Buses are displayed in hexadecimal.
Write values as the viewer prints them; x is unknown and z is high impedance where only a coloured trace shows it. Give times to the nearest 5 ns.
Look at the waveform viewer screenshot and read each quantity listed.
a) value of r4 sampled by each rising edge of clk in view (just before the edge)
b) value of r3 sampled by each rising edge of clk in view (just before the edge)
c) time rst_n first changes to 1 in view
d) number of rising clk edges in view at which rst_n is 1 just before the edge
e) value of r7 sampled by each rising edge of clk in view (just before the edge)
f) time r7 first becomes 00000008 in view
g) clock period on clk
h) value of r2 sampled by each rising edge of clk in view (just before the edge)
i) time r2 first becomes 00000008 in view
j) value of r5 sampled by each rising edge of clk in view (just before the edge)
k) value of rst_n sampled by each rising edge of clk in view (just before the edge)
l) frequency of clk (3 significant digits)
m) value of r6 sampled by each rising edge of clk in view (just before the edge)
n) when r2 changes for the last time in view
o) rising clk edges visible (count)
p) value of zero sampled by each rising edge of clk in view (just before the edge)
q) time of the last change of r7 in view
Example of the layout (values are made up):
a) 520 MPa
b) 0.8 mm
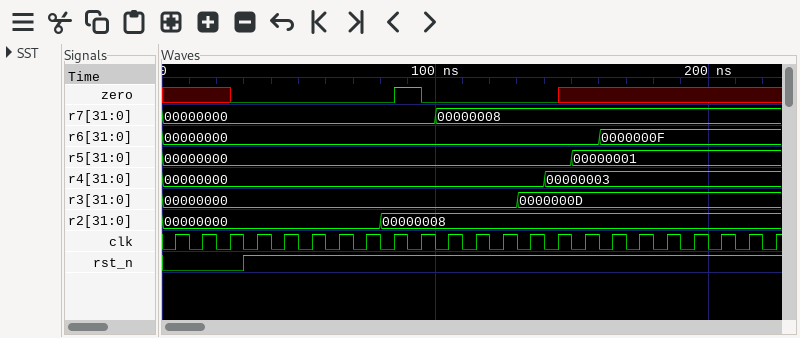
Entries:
a) 00000000, 00000000, 00000000, 00000000, 00000000, 00000000, 00000000, 00000000, 00000000, 00000000, 00000000, 00000000, 00000000, 00000000, 00000003, 00000003, 00000003, 00000003, 00000003, 00000003, 00000003, 00000003, 00000003
b) 00000000, 00000000, 00000000, 00000000, 00000000, 00000000, 00000000, 00000000, 00000000, 00000000, 00000000, 00000000, 00000000, 0000000D, 0000000D, 0000000D, 0000000D, 0000000D, 0000000D, 0000000D, 0000000D, 0000000D, 0000000D
c) 30 ns
d) 20
e) 00000000, 00000000, 00000000, 00000000, 00000000, 00000000, 00000000, 00000000, 00000000, 00000000, 00000008, 00000008, 00000008, 00000008, 00000008, 00000008, 00000008, 00000008, 00000008, 00000008, 00000008, 00000008, 00000008
f) 100 ns
g) 10 ns
h) 00000000, 00000000, 00000000, 00000000, 00000000, 00000000, 00000000, 00000000, 00000008, 00000008, 00000008, 00000008, 00000008, 00000008, 00000008, 00000008, 00000008, 00000008, 00000008, 00000008, 00000008, 00000008, 00000008
i) 80 ns
j) 00000000, 00000000, 00000000, 00000000, 00000000, 00000000, 00000000, 00000000, 00000000, 00000000, 00000000, 00000000, 00000000, 00000000, 00000000, 00000001, 00000001, 00000001, 00000001, 00000001, 00000001, 00000001, 00000001
k) 0 0 0 1 1 1 1 1 1 1 1 1 1 1 1 1 1 1 1 1 1 1 1
l) 100 MHz
m) 00000000, 00000000, 00000000, 00000000, 00000000, 00000000, 00000000, 00000000, 00000000, 00000000, 00000000, 00000000, 00000000, 00000000, 00000000, 00000000, 0000000F, 0000000F, 0000000F, 0000000F, 0000000F, 0000000F, 0000000F
n) 80 ns
o) 23
p) x x x 0 0 0 0 0 0 1 0 0 0 0 0 x x x x x x x x
q) 100 ns
